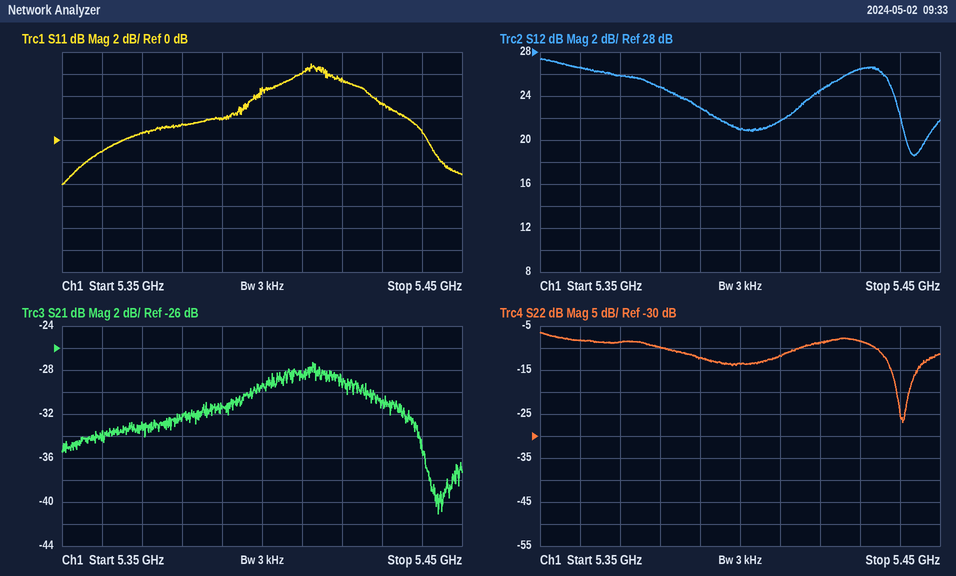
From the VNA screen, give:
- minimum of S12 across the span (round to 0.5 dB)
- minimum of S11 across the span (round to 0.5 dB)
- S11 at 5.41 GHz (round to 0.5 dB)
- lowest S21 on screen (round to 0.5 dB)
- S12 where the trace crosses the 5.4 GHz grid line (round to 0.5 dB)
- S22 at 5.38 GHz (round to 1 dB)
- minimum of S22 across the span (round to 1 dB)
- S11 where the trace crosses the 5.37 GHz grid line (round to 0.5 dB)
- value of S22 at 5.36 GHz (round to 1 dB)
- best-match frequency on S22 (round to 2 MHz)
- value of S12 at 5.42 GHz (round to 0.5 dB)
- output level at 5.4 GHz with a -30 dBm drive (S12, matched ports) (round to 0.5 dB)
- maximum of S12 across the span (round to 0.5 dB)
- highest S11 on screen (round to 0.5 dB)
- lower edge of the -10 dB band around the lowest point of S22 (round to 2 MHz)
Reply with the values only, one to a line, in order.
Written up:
18.5 dB
-4.0 dB
6.0 dB
-41.0 dB
21.0 dB
-10 dB
-27 dB
0.5 dB
-8 dB
5.440 GHz
24.5 dB
-9.0 dBm
27.5 dB
7.0 dB
5.434 GHz
